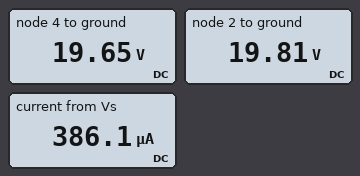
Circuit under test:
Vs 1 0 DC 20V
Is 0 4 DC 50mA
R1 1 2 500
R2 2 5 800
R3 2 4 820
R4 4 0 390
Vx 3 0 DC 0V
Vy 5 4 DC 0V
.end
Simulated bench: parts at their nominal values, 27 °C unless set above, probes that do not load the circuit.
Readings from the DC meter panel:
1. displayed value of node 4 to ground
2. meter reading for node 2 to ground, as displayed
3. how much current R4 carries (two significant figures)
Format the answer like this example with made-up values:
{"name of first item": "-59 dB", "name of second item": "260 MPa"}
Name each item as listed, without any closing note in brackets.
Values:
{"displayed value of node 4 to ground": "19.65 V", "meter reading for node 2 to ground, as displayed": "19.81 V", "how much current R4 carries": "50 mA"}
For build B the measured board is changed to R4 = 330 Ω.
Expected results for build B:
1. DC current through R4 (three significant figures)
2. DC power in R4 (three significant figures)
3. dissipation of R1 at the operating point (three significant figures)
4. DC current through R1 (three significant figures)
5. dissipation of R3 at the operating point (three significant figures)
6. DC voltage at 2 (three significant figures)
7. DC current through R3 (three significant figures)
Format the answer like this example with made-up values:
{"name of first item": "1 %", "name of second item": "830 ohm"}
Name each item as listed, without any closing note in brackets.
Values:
{"DC current through R4": "52.8 mA", "DC power in R4": "921 mW", "dissipation of R1 at the operating point": "4.02 mW", "DC current through R1": "2.83 mA", "dissipation of R3 at the operating point": "1.61 mW", "DC voltage at 2": "18.6 V", "DC current through R3": "1.40 mA"}
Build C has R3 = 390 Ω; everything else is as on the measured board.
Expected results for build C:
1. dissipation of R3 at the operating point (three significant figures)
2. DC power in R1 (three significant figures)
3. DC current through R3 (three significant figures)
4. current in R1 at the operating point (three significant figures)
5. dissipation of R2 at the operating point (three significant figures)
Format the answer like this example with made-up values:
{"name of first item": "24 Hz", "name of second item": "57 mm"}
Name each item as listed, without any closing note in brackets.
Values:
{"dissipation of R3 at the operating point": "33.2 µW", "DC power in R1": "94.2 µW", "DC current through R3": "292 µA", "current in R1 at the operating point": "434 µA", "dissipation of R2 at the operating point": "16.2 µW"}
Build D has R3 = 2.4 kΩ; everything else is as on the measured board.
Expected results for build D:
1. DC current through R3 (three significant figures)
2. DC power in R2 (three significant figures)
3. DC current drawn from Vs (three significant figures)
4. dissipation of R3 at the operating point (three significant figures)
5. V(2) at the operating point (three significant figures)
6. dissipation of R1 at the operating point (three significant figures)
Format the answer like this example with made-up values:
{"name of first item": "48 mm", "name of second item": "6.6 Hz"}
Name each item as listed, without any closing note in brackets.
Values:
{"DC current through R3": "83.9 µA", "DC power in R2": "50.7 µW", "DC current drawn from Vs": "336 µA", "dissipation of R3 at the operating point": "16.9 µW", "V(2) at the operating point": "19.8 V", "dissipation of R1 at the operating point": "56.3 µW"}
